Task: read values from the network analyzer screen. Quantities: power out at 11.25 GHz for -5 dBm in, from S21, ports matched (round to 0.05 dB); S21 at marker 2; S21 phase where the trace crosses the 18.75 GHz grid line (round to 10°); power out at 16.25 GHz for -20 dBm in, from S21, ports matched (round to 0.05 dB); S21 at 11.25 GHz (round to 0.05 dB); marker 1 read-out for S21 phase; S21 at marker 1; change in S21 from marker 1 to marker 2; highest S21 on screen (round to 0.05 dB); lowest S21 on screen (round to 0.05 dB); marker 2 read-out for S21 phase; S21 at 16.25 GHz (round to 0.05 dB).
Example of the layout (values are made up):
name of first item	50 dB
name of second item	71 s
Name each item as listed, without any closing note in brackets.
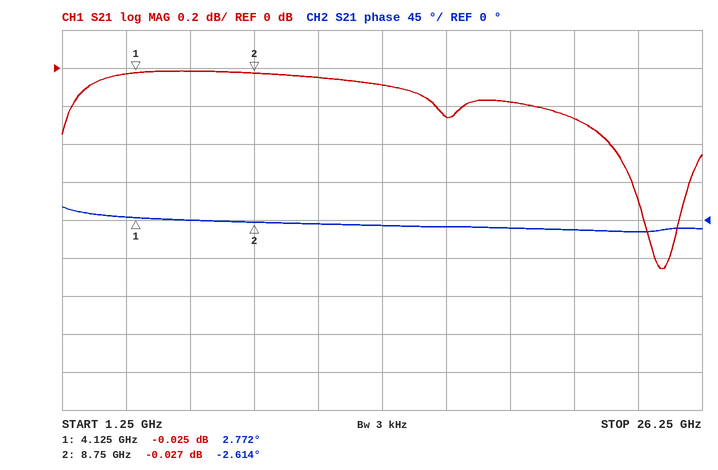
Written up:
power out at 11.25 GHz for -5 dBm in, from S21, ports matched	-5.05 dBm
S21 at marker 2	-0.027 dB
S21 phase where the trace crosses the 18.75 GHz grid line	-10°
power out at 16.25 GHz for -20 dBm in, from S21, ports matched	-20.25 dBm
S21 at 11.25 GHz	-0.05 dB
marker 1 read-out for S21 phase	2.772°
S21 at marker 1	-0.025 dB
change in S21 from marker 1 to marker 2	-0.002 dB
highest S21 on screen	0.00 dB
lowest S21 on screen	-1.05 dB
marker 2 read-out for S21 phase	-2.614°
S21 at 16.25 GHz	-0.25 dB
